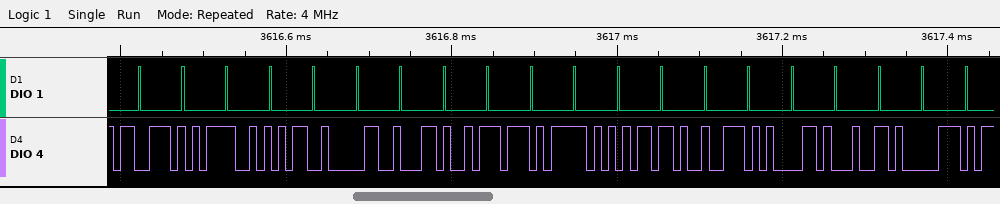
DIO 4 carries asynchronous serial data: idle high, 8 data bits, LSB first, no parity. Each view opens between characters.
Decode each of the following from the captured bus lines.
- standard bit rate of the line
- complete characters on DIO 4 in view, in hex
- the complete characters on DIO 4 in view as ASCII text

115200 baud
73, 3D, 35, 30, 2C, 77, 5F, 6D, 72, 61, 64, 70
"s=50,w_mradp"
